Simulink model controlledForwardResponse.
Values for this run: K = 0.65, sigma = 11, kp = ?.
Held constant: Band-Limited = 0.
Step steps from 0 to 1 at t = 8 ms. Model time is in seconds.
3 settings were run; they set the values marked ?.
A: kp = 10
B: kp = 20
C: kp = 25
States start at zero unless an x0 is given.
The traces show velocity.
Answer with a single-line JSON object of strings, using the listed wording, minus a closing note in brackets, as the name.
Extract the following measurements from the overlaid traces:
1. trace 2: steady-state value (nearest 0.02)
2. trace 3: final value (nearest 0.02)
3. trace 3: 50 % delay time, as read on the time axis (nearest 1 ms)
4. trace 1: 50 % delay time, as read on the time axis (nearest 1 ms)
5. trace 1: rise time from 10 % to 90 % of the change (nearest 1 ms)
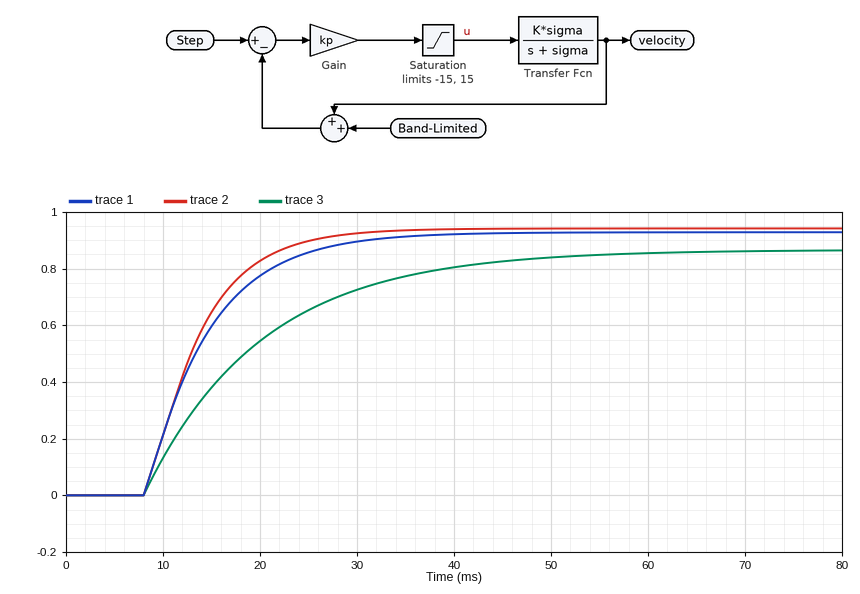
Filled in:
{"trace 2: steady-state value": "0.94", "trace 3: final value": "0.86", "trace 3: 50 % delay time, as read on the time axis": "16 ms", "trace 1: 50 % delay time, as read on the time axis": "13 ms", "trace 1: rise time from 10 % to 90 % of the change": "14 ms"}
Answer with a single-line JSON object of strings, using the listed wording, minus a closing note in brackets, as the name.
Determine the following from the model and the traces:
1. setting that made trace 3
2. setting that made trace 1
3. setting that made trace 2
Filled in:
{"setting that made trace 3": "A", "setting that made trace 1": "B", "setting that made trace 2": "C"}
